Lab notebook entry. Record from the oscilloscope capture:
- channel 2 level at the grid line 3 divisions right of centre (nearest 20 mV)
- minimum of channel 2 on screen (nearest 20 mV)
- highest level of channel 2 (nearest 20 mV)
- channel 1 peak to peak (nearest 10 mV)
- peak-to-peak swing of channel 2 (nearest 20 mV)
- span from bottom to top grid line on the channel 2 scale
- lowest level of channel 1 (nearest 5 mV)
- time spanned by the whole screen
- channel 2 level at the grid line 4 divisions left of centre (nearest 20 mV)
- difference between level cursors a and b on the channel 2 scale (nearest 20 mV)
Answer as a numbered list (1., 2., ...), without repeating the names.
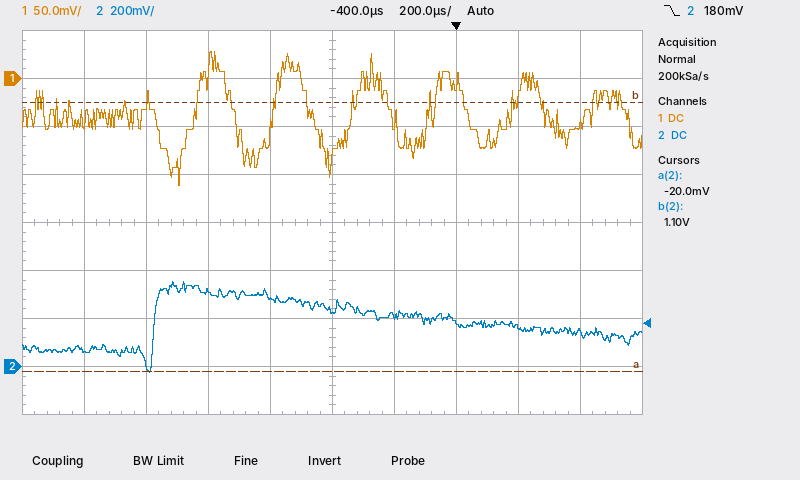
1. 160 mV
2. -20 mV
3. 360 mV
4. 140 mV
5. 380 mV
6. 1.6 V
7. -110 mV
8. 2 ms
9. 60 mV
10. 1.12 V
